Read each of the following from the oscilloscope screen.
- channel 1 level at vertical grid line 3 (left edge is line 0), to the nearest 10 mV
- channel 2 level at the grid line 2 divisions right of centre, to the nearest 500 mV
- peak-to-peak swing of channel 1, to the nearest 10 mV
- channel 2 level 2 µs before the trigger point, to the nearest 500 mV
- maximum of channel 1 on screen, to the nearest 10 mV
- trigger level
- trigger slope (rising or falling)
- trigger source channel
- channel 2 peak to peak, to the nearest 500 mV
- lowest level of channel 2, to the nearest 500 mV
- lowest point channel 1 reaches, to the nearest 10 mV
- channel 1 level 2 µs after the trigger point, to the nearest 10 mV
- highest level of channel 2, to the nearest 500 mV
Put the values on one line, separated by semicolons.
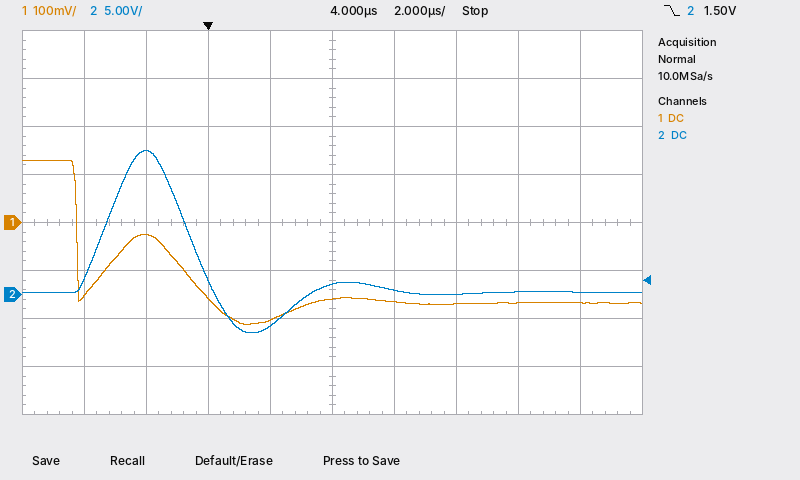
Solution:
-160 mV; 0.0 V; 340 mV; 15.0 V; 130 mV; 1.50 V; falling; channel 2; 19.0 V; -4.0 V; -210 mV; -200 mV; 15.0 V
